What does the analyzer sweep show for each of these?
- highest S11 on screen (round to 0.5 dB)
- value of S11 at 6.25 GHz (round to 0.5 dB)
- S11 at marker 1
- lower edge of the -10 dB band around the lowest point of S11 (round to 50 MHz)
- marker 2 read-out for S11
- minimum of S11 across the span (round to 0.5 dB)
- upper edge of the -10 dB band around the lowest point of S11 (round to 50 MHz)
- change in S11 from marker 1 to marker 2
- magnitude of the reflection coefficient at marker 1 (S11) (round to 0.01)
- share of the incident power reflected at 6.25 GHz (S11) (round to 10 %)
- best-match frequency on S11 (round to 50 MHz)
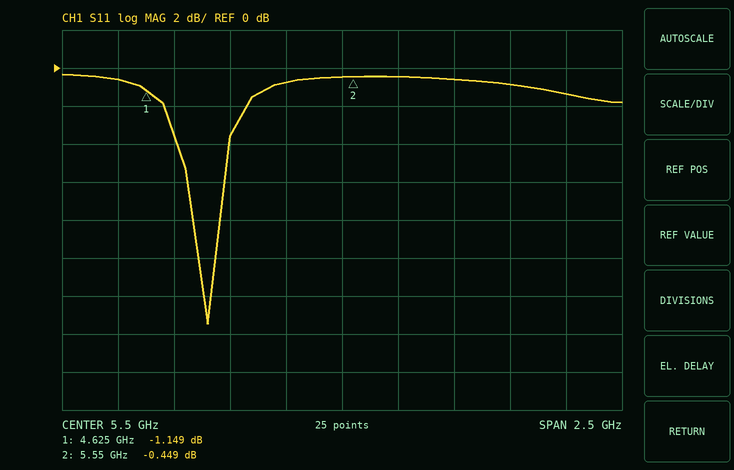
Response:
-0.5 dB
-1.0 dB
-1.149 dB
4.85 GHz
-0.449 dB
-13.5 dB
4.95 GHz
0.700 dB
0.88
80 %
4.90 GHz
